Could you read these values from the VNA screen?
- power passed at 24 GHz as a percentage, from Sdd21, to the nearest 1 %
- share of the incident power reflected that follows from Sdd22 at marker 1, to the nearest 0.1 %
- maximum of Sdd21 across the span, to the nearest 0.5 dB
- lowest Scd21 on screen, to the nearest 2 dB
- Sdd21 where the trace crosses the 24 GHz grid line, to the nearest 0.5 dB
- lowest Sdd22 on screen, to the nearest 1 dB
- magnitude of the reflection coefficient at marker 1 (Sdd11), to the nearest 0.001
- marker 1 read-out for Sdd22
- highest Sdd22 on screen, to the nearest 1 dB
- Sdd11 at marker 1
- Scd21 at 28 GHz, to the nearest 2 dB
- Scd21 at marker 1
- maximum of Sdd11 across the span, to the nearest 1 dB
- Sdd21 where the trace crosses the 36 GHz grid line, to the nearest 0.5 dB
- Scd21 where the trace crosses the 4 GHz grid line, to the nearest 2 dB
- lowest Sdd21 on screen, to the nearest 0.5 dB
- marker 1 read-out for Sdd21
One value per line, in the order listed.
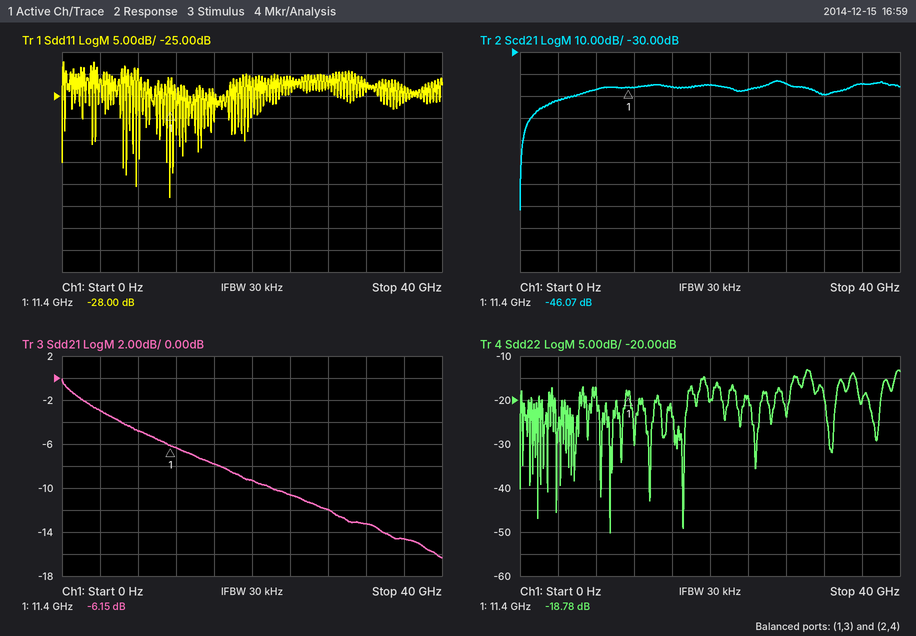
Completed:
9 %
1.3 %
0.0 dB
-102 dB
-10.5 dB
-50 dB
0.040
-18.78 dB
-13 dB
-28.00 dB
-44 dB
-46.07 dB
-17 dB
-14.5 dB
-52 dB
-16.5 dB
-6.15 dB
